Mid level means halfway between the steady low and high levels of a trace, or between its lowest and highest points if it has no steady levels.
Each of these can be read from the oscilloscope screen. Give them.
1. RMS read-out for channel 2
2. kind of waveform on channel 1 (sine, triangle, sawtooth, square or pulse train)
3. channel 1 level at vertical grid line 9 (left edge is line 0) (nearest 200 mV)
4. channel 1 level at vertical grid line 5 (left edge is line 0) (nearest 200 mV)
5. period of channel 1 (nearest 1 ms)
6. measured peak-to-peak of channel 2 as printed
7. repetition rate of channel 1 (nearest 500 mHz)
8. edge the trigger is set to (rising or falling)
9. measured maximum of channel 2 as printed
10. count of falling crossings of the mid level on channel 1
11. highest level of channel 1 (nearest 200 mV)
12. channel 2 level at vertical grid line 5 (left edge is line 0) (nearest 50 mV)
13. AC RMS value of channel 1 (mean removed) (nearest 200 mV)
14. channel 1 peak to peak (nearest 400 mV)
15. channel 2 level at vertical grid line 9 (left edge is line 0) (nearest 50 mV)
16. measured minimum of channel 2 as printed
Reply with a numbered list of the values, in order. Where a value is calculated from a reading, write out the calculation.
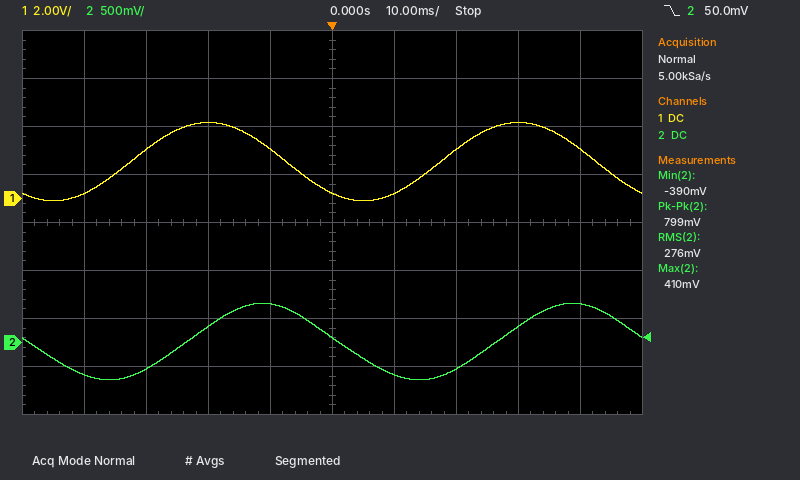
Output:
1. 276 mV
2. sine
3. 2.0 V
4. 200 mV
5. 50 ms
6. 799 mV
7. 1 / 50 ms ≈ 20.0 Hz
8. falling
9. 410 mV
10. 2
11. 3.2 V
12. 50 mV
13. 3.2 V / (2√2) ≈ 1.13 V, so 1.2 V to the nearest 200 mV
14. 3.2 V
15. 400 mV
16. -390 mV
